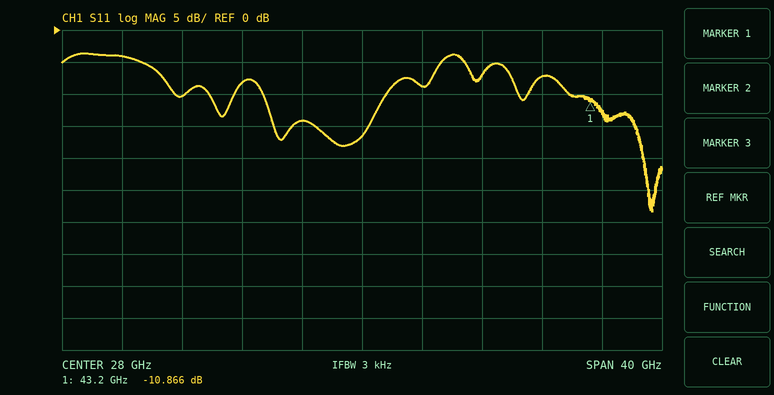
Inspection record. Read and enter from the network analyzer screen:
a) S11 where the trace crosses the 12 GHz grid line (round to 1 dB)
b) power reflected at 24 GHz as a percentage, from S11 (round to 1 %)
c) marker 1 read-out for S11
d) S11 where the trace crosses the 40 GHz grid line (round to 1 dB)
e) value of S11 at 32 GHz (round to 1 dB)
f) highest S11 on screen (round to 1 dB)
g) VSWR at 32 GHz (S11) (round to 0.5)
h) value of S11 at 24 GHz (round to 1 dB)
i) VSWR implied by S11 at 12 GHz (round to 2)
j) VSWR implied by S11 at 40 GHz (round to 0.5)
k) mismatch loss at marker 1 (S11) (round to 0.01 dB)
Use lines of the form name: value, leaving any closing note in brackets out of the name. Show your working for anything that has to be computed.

S11 where the trace crosses the 12 GHz grid line: -4 dB
power reflected at 24 GHz as a percentage, from S11: 10^(-14/10) ≈ 4 %
marker 1 read-out for S11: -10.866 dB
S11 where the trace crosses the 40 GHz grid line: -7 dB
value of S11 at 32 GHz: -9 dB
highest S11 on screen: -4 dB
VSWR at 32 GHz (S11): |Γ| = 10^(-9/20) = 0.3548; VSWR = (1 + 0.3548)/(1 − 0.3548) ≈ 2.10, so 2.0 to the nearest 0.5
value of S11 at 24 GHz: -14 dB
VSWR implied by S11 at 12 GHz: |Γ| = 10^(-4/20) = 0.6310; VSWR = (1 + 0.6310)/(1 − 0.6310) ≈ 4
VSWR implied by S11 at 40 GHz: |Γ| = 10^(-7/20) = 0.4467; VSWR = (1 + 0.4467)/(1 − 0.4467) ≈ 2.61, so 2.5 to the nearest 0.5
mismatch loss at marker 1 (S11): −10 log10(1 − 10^(-10.866/10)) ≈ 0.37 dB
